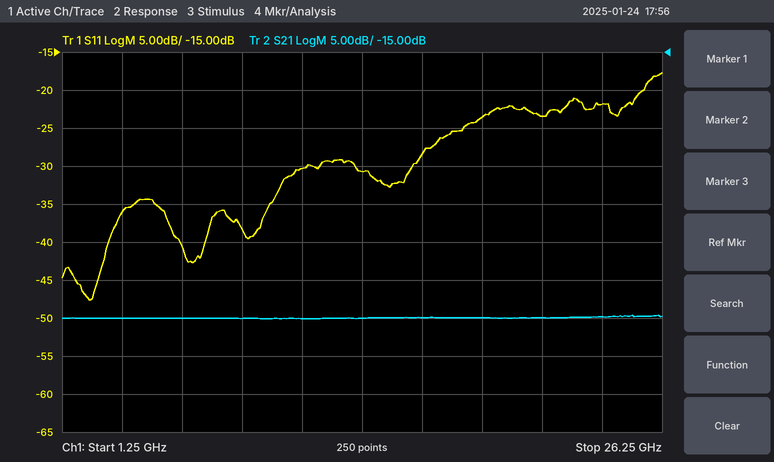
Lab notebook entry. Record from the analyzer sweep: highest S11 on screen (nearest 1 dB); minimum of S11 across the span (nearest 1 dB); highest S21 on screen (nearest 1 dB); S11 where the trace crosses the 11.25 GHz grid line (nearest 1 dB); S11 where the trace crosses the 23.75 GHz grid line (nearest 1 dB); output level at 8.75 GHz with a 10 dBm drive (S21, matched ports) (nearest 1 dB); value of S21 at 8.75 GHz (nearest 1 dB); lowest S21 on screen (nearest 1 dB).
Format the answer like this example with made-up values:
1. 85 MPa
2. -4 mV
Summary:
1. -18 dB
2. -48 dB
3. -50 dB
4. -30 dB
5. -22 dB
6. -40 dBm
7. -50 dB
8. -50 dB
